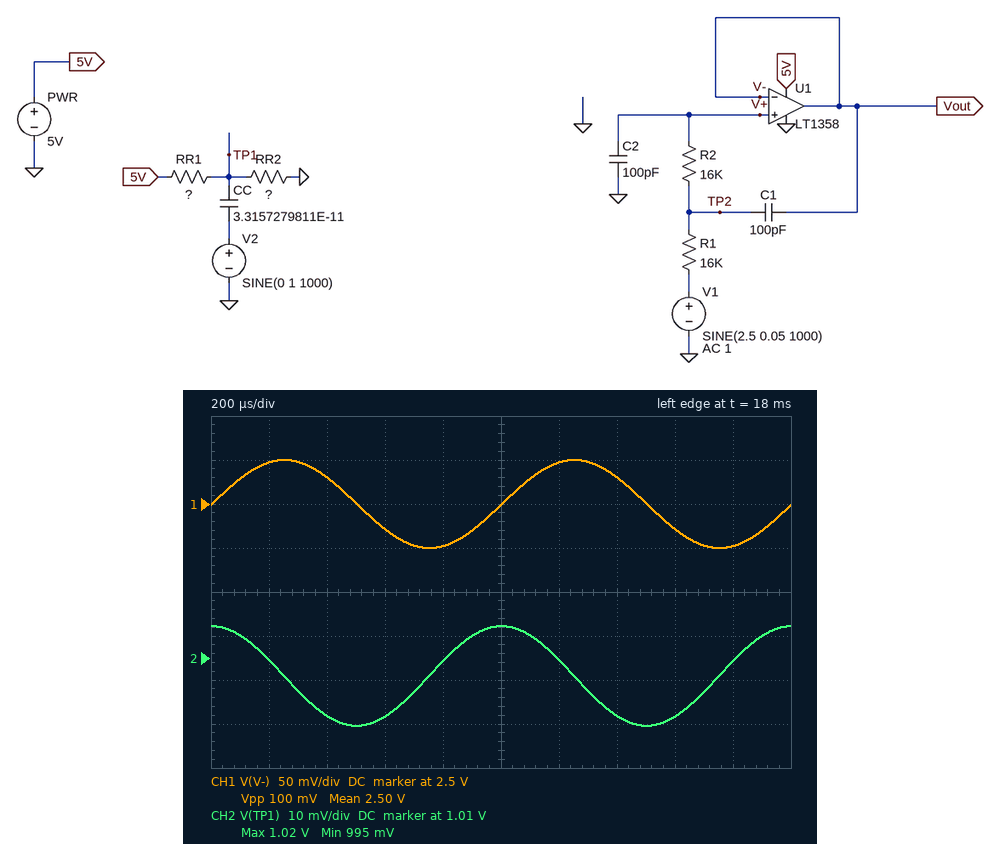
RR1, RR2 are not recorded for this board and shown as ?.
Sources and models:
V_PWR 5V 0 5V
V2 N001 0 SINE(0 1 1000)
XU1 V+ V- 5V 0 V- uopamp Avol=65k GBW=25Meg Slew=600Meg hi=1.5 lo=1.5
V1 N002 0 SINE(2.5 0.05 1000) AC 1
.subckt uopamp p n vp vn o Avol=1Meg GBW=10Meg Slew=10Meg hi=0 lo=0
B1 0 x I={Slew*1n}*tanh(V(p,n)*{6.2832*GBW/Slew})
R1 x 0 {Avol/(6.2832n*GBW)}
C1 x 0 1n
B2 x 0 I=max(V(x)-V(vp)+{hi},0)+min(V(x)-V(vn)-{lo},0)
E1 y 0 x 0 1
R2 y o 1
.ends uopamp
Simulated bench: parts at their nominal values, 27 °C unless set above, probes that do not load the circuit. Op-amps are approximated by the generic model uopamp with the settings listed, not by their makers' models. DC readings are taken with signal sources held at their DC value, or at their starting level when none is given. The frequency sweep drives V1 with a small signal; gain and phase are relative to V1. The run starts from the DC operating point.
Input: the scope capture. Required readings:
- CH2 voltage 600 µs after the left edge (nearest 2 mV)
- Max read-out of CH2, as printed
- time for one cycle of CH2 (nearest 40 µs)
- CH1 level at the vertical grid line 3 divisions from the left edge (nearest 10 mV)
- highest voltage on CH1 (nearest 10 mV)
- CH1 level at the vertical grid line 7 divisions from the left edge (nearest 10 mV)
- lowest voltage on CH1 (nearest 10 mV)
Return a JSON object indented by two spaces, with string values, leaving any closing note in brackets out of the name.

{
  "CH2 voltage 600 µs after the left edge": "996 mV",
  "Max read-out of CH2, as printed": "1.02 V",
  "time for one cycle of CH2": "1.00 ms",
  "CH1 level at the vertical grid line 3 divisions from the left edge": "2.47 V",
  "highest voltage on CH1": "2.55 V",
  "CH1 level at the vertical grid line 7 divisions from the left edge": "2.53 V",
  "lowest voltage on CH1": "2.45 V"
}
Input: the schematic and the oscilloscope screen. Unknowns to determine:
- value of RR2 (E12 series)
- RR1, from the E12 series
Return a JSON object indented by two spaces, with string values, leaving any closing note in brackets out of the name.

{
  "value of RR2": "68 kΩ",
  "RR1, from the E12 series": "270 kΩ"
}
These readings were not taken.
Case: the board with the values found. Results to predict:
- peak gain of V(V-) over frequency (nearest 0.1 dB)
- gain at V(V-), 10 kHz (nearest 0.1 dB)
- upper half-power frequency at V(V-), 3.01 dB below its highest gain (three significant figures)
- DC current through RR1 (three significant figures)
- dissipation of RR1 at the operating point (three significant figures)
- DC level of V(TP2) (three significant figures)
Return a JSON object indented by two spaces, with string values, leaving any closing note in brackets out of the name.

{
  "peak gain of V(V-) over frequency": "0 dB",
  "gain at V(V-), 10 kHz": "-0.1 dB",
  "upper half-power frequency at V(V-), 3.01 dB below its highest gain": "64.1 kHz",
  "DC current through RR1": "14.8 µA",
  "dissipation of RR1 at the operating point": "59.1 µW",
  "DC level of V(TP2)": "2.50 V"
}
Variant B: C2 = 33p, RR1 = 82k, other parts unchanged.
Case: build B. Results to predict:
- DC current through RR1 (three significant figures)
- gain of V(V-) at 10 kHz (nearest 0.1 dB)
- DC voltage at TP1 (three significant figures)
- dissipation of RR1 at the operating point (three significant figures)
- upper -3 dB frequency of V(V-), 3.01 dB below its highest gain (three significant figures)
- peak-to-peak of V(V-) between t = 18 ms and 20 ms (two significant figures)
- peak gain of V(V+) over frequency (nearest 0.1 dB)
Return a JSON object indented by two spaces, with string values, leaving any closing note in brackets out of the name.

{
  "DC current through RR1": "33.3 µA",
  "gain of V(V-) at 10 kHz": "0 dB",
  "DC voltage at TP1": "2.27 V",
  "dissipation of RR1 at the operating point": "91.1 µW",
  "upper -3 dB frequency of V(V-), 3.01 dB below its highest gain": "195 kHz",
  "peak-to-peak of V(V-) between t = 18 ms and 20 ms": "100 mV",
  "peak gain of V(V+) over frequency": "0.6 dB"
}
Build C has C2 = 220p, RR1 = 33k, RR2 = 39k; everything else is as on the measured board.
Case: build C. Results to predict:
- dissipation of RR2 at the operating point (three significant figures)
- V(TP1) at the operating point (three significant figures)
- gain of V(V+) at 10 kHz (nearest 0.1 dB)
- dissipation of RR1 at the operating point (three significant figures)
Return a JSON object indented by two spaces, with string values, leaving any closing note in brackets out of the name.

{
  "dissipation of RR2 at the operating point": "188 µW",
  "V(TP1) at the operating point": "2.71 V",
  "gain of V(V+) at 10 kHz": "-0.6 dB",
  "dissipation of RR1 at the operating point": "159 µW"
}
